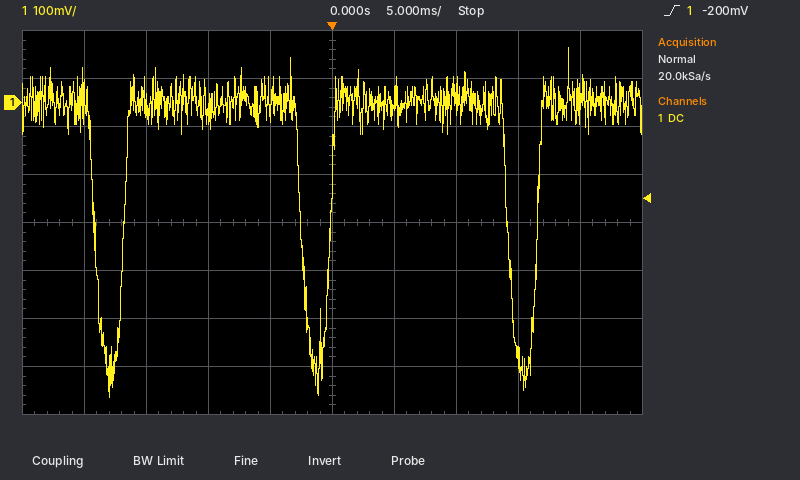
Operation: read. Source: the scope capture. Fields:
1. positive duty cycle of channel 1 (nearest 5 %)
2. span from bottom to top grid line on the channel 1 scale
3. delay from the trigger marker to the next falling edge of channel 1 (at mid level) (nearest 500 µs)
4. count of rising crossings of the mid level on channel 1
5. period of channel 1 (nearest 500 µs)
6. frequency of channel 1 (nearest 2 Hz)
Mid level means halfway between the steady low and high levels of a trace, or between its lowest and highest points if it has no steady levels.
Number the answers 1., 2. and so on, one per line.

1. 85 %
2. 800 mV
3. 14.0 ms
4. 3
5. 16.5 ms
6. 60 Hz
